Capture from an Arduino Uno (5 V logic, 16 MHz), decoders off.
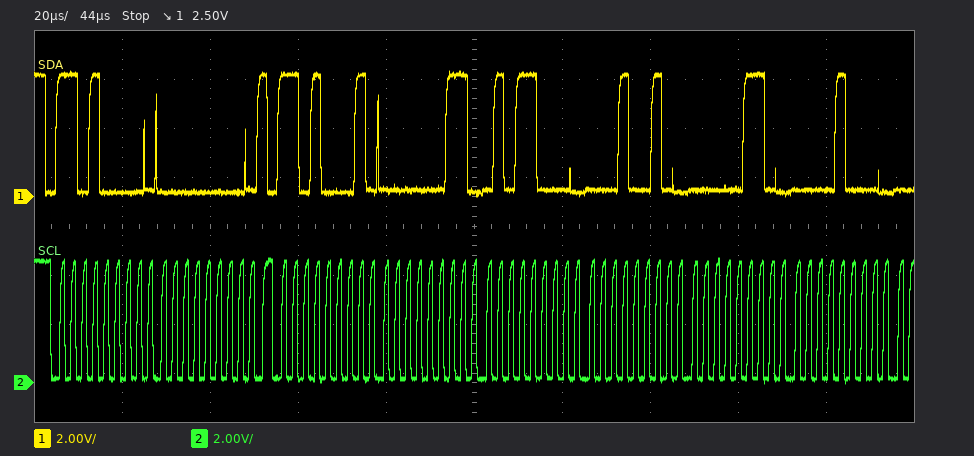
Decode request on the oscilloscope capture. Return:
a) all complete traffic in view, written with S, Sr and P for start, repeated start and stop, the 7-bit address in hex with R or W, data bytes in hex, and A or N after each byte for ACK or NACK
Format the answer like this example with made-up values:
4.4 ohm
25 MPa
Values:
S 68W A 00 A Sr 68R A 03 A 58 A 12 A 06 A 08 A
